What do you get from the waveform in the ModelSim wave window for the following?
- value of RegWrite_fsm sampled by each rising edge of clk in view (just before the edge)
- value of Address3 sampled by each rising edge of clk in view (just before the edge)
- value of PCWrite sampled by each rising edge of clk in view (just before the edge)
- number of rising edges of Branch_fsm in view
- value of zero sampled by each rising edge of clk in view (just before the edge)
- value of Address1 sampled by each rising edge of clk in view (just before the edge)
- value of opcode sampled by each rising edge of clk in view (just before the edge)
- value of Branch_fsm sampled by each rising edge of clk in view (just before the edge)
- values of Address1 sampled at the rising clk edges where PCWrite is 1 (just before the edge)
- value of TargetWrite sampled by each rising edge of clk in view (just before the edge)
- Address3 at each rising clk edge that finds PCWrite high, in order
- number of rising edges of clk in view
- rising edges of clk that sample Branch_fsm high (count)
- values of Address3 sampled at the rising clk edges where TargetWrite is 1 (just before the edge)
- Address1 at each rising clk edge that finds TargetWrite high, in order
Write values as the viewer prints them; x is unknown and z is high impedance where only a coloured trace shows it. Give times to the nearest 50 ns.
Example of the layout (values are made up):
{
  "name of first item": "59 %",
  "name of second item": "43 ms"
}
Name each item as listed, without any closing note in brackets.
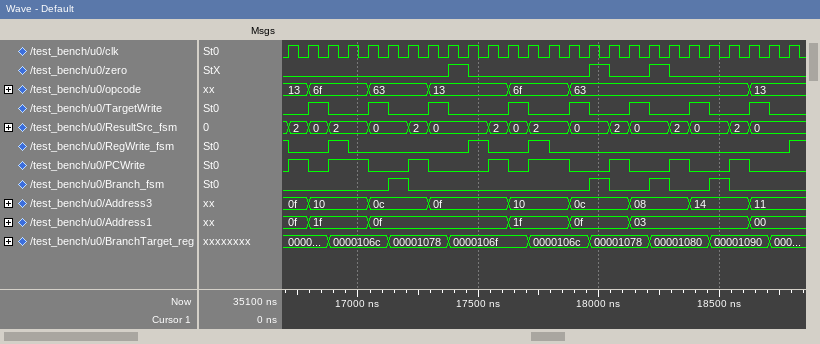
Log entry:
{
  "value of RegWrite_fsm sampled by each rising edge of clk in view": "1 0 0 1 0 0 0 0 0 0 1 0 0 1 0 0 0 0 0 0 0 0 0 0 0 0",
  "value of Address3 sampled by each rising edge of clk in view": "0f, 0f, 10, 10, 10, 0c, 0c, 0c, 0f, 0f, 0f, 0f, 10, 10, 10, 0c, 0c, 0c, 08, 08, 08, 14, 14, 14, 11, 11",
  "value of PCWrite sampled by each rising edge of clk in view": "0 1 0 1 1 0 0 1 0 0 0 1 0 1 1 0 0 1 0 0 1 0 0 1 0 0",
  "number of rising edges of Branch_fsm in view": "4",
  "value of zero sampled by each rising edge of clk in view": "0 0 0 0 0 0 0 0 0 1 0 0 0 0 0 0 1 0 0 1 0 0 0 0 0 0",
  "value of Address1 sampled by each rising edge of clk in view": "0f, 0f, 1f, 1f, 1f, 0f, 0f, 0f, 0f, 0f, 0f, 0f, 1f, 1f, 1f, 0f, 0f, 0f, 03, 03, 03, 03, 03, 03, 00, 00",
  "value of opcode sampled by each rising edge of clk in view": "13, 13, 6f, 6f, 6f, 63, 63, 63, 13, 13, 13, 13, 6f, 6f, 6f, 63, 63, 63, 63, 63, 63, 63, 63, 63, 13, 13",
  "value of Branch_fsm sampled by each rising edge of clk in view": "0 0 0 0 0 0 1 0 0 0 0 0 0 0 0 0 1 0 0 1 0 0 1 0 0 0",
  "values of Address1 sampled at the rising clk edges where PCWrite is 1": "0f, 1f, 1f, 0f, 0f, 1f, 1f, 0f, 03, 03",
  "value of TargetWrite sampled by each rising edge of clk in view": "0 0 1 0 0 1 0 0 1 0 0 0 1 0 0 1 0 0 1 0 0 1 0 0 1 0",
  "Address3 at each rising clk edge that finds PCWrite high, in order": "0f, 10, 10, 0c, 0f, 10, 10, 0c, 08, 14",
  "number of rising edges of clk in view": "26",
  "rising edges of clk that sample Branch_fsm high": "4",
  "values of Address3 sampled at the rising clk edges where TargetWrite is 1": "10, 0c, 0f, 10, 0c, 08, 14, 11",
  "Address1 at each rising clk edge that finds TargetWrite high, in order": "1f, 0f, 0f, 1f, 0f, 03, 03, 00"
}
